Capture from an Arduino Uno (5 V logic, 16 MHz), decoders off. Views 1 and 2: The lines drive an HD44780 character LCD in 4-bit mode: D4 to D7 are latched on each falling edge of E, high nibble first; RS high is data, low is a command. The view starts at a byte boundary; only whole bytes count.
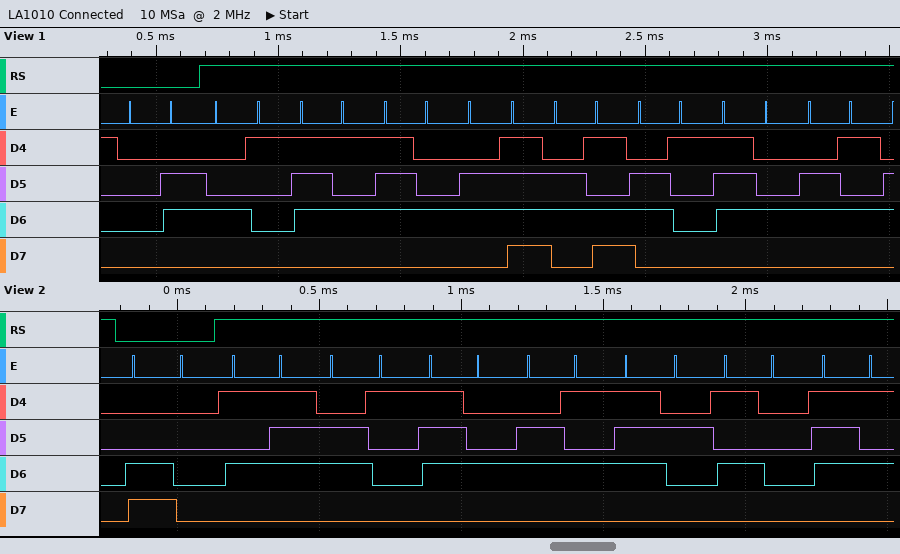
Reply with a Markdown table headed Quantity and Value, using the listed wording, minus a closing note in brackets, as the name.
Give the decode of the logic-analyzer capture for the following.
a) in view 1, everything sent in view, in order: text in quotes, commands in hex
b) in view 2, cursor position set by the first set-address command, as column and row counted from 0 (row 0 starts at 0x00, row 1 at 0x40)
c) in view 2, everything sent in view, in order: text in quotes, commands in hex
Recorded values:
| Quantity | Value |
|---|---|
| in view 1, everything sent in view, in order: text in quotes, commands in hex | 0x06 "Automate" |
| in view 2, cursor position set by the first set-address command, as column and row counted from 0 | column 0, row 1 |
| in view 2, everything sent in view, in order: text in quotes, commands in hex | 0xC0 "WaterPu" |
